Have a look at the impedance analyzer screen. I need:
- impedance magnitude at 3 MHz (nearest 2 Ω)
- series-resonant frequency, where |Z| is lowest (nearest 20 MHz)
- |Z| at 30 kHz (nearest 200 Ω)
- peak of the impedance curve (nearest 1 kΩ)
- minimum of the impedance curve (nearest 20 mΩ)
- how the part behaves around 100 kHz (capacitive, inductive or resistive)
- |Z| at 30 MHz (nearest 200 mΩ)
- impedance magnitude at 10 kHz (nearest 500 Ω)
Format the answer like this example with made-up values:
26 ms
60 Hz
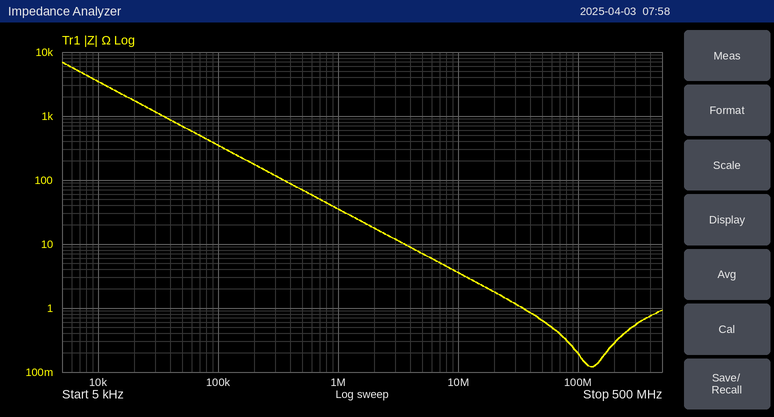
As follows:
12 Ω
120 MHz
1.2 kΩ
7 kΩ
120 mΩ
capacitive
1.2 Ω
3.5 kΩ
